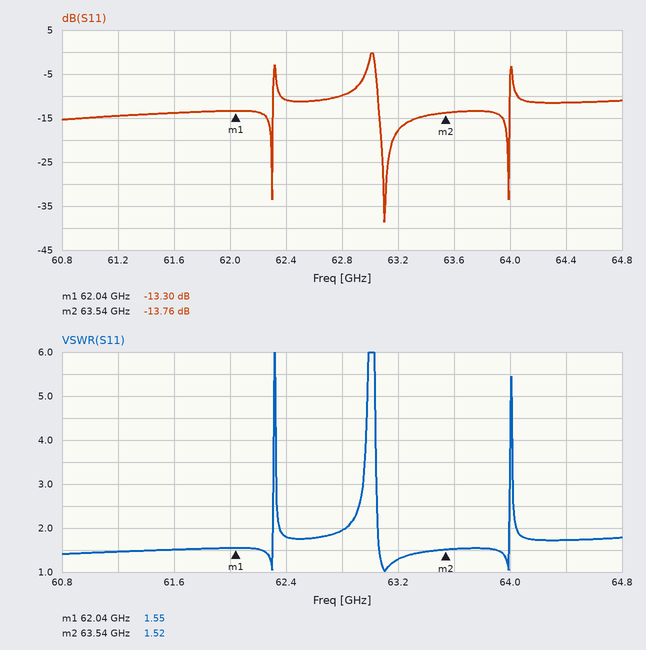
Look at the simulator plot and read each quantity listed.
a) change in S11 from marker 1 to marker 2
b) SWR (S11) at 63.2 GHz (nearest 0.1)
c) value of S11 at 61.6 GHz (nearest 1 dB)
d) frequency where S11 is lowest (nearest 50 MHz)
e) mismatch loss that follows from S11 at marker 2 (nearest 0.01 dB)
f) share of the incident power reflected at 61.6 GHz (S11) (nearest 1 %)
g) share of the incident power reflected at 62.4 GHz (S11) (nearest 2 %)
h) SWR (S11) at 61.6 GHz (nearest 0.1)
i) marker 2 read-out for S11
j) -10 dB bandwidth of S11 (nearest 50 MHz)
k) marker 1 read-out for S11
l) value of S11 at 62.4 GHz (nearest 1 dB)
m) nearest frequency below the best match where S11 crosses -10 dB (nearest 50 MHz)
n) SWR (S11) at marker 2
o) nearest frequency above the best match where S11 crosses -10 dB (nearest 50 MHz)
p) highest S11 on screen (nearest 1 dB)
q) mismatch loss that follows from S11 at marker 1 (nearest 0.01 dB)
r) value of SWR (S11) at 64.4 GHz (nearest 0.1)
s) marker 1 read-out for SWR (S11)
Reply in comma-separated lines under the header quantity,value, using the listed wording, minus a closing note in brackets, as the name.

quantity,value
change in S11 from marker 1 to marker 2,-0.46 dB
SWR (S11) at 63.2 GHz,1.3
value of S11 at 61.6 GHz,-14 dB
frequency where S11 is lowest,63.10 GHz
mismatch loss that follows from S11 at marker 2,0.19 dB
share of the incident power reflected at 61.6 GHz (S11),4 %
share of the incident power reflected at 62.4 GHz (S11),8 %
SWR (S11) at 61.6 GHz,1.5
marker 2 read-out for S11,-13.76 dB
-10 dB bandwidth of S11,950 MHz
marker 1 read-out for S11,-13.30 dB
value of S11 at 62.4 GHz,-11 dB
nearest frequency below the best match where S11 crosses -10 dB,63.05 GHz
SWR (S11) at marker 2,1.52
nearest frequency above the best match where S11 crosses -10 dB,64.00 GHz
highest S11 on screen,0 dB
mismatch loss that follows from S11 at marker 1,0.21 dB
value of SWR (S11) at 64.4 GHz,1.7
marker 1 read-out for SWR,1.55
